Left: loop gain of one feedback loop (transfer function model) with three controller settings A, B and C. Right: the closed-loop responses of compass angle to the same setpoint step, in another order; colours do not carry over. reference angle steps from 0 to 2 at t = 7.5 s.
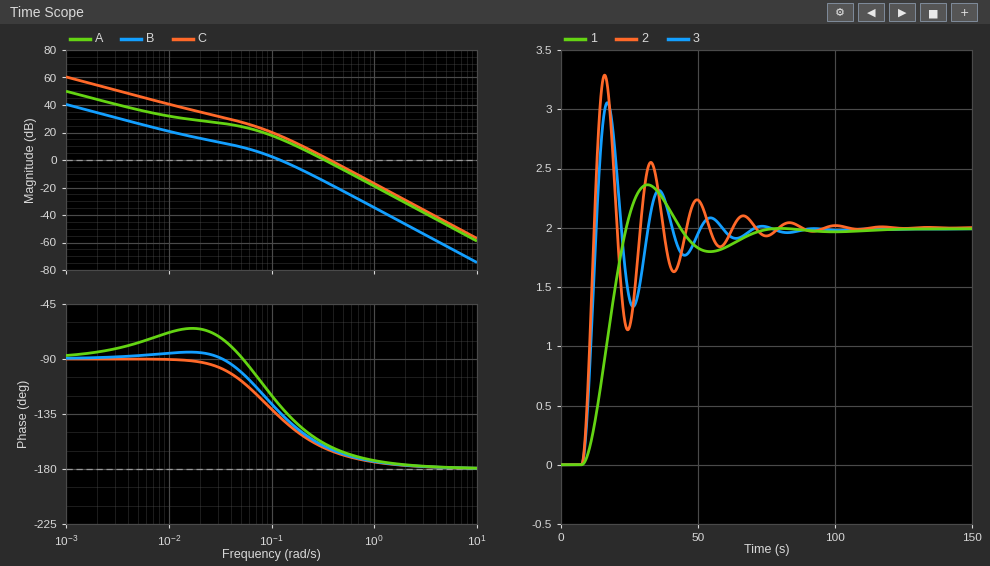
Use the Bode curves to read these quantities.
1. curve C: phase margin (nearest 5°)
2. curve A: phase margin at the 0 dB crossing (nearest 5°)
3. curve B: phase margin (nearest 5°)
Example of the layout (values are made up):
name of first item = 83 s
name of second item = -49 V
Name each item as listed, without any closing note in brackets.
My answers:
curve C: phase margin = 15°
curve A: phase margin at the 0 dB crossing = 20°
curve B: phase margin = 45°
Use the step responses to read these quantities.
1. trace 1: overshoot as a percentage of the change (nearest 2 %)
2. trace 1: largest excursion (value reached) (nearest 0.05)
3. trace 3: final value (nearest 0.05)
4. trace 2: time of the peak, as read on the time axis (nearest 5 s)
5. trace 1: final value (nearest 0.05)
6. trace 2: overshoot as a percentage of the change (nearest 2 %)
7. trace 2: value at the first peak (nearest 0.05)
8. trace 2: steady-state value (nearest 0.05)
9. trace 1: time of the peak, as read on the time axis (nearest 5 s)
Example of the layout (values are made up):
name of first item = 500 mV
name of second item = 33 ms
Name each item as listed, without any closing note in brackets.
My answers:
trace 1: overshoot as a percentage of the change = 18 %
trace 1: largest excursion (value reached) = 2.35
trace 3: final value = 2.00
trace 2: time of the peak, as read on the time axis = 15 s
trace 1: final value = 2.00
trace 2: overshoot as a percentage of the change = 64 %
trace 2: value at the first peak = 3.30
trace 2: steady-state value = 2.00
trace 1: time of the peak, as read on the time axis = 30 s
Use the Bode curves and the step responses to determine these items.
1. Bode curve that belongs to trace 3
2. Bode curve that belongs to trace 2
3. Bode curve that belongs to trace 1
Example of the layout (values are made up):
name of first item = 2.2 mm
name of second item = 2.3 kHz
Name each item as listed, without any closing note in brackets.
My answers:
Bode curve that belongs to trace 3 = A
Bode curve that belongs to trace 2 = C
Bode curve that belongs to trace 1 = B
